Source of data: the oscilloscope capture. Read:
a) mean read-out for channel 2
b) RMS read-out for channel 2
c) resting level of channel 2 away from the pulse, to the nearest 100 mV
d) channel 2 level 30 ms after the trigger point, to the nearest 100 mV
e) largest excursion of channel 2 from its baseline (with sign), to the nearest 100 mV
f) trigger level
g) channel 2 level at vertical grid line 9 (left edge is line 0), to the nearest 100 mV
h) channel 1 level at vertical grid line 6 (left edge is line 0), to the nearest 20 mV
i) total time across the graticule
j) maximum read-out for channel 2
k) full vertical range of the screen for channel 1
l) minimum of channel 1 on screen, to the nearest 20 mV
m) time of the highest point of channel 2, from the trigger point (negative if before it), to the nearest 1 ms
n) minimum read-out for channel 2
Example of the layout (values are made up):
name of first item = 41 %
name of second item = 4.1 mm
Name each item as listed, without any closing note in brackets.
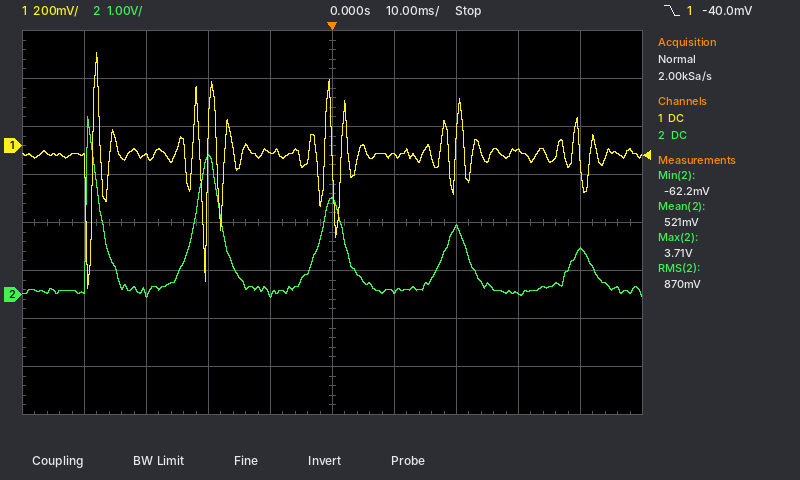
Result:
mean read-out for channel 2 = 521 mV
RMS read-out for channel 2 = 870 mV
resting level of channel 2 away from the pulse, to the nearest 100 mV = 100 mV
channel 2 level 30 ms after the trigger point, to the nearest 100 mV = 0.0 V
largest excursion of channel 2 from its baseline (with sign), to the nearest 100 mV = +3.6 V
trigger level = -40.0 mV
channel 2 level at vertical grid line 9 (left edge is line 0), to the nearest 100 mV = 900 mV
channel 1 level at vertical grid line 6 (left edge is line 0), to the nearest 20 mV = -40 mV
total time across the graticule = 100 ms
maximum read-out for channel 2 = 3.71 V
full vertical range of the screen for channel 1 = 1.6 V
minimum of channel 1 on screen, to the nearest 20 mV = -600 mV
time of the highest point of channel 2, from the trigger point (negative if before it), to the nearest 1 ms = -39 ms
minimum read-out for channel 2 = -62.2 mV
